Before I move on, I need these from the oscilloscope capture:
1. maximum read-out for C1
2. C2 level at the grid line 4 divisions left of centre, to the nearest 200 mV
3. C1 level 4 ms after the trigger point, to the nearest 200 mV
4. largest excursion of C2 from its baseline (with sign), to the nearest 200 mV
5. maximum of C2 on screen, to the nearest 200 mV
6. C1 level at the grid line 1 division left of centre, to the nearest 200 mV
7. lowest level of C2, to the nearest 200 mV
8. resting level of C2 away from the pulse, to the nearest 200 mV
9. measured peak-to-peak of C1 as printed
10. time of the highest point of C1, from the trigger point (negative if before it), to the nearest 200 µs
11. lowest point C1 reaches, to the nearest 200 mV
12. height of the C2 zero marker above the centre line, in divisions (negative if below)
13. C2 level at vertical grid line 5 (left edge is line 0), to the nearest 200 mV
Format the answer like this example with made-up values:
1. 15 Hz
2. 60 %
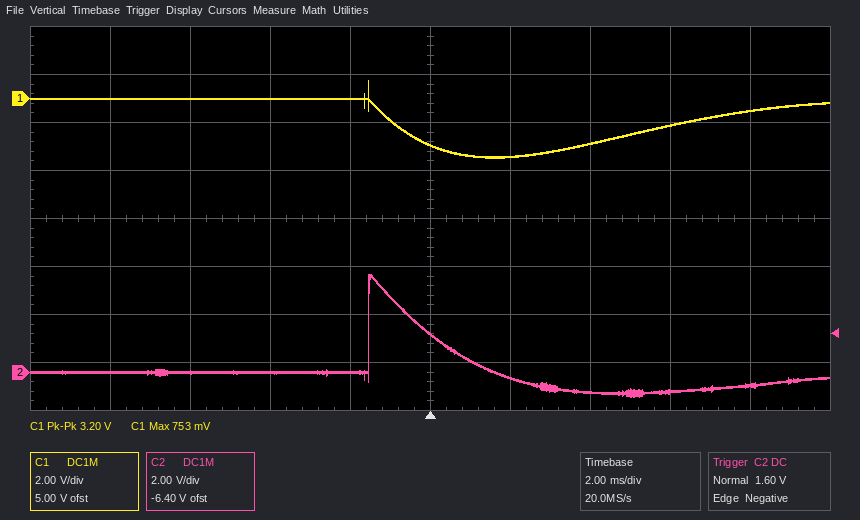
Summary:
1. 753 mV
2. 0.0 V
3. -1.8 V
4. +4.0 V
5. 4.0 V
6. 0.0 V
7. -1.0 V
8. 0.0 V
9. 3.20 V
10. -1.6 ms
11. -2.4 V
12. -3.2 div
13. 1.6 V
